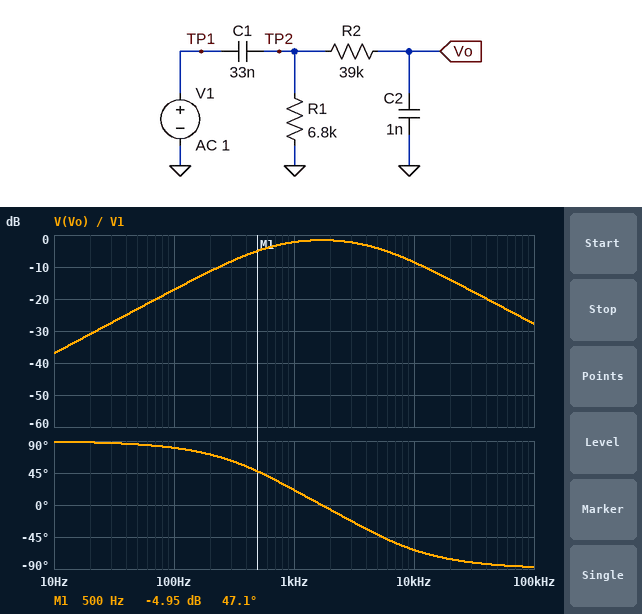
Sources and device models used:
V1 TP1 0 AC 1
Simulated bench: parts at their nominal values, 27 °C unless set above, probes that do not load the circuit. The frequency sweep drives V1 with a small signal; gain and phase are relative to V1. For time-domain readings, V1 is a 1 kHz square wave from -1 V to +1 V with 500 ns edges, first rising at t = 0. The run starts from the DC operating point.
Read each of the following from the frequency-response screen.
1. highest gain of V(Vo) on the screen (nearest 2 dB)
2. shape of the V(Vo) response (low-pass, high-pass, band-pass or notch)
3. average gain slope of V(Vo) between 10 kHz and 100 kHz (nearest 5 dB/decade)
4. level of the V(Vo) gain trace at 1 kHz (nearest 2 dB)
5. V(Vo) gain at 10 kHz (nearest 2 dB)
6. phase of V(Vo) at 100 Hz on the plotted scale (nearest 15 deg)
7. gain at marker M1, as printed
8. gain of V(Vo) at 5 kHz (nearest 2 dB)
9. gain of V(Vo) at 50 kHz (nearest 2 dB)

-2 dB
band-pass
-20 dB/decade
-2 dB
-8 dB
75 deg
-4.95 dB
-4 dB
-22 dB
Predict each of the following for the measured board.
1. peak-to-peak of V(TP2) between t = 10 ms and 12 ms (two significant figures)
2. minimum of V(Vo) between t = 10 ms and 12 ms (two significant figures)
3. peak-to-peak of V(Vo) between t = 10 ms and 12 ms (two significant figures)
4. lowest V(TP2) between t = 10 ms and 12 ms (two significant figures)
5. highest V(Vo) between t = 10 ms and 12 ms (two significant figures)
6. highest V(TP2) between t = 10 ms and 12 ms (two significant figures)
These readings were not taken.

3.6 V
-1.2 V
2.4 V
-1.8 V
1.2 V
1.8 V
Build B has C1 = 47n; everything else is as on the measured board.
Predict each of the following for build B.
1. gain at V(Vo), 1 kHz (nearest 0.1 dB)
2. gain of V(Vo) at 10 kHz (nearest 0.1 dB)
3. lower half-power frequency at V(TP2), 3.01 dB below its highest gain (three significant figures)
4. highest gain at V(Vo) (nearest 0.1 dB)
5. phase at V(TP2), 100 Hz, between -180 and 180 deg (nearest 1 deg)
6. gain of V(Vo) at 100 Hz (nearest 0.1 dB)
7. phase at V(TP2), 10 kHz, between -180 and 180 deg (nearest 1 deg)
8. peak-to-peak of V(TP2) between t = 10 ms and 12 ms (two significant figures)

-1.4 dB
-8.5 dB
510 Hz
-1.2 dB
78 deg
-14.1 dB
3 deg
3.3 V
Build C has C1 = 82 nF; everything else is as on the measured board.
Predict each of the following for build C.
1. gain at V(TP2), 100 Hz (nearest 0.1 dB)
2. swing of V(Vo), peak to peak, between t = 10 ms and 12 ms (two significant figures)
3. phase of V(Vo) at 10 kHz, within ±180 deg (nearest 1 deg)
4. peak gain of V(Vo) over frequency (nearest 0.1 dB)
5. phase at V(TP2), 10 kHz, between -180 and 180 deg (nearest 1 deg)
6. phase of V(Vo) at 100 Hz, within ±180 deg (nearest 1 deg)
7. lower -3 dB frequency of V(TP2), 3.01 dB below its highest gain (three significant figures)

-9.6 dB
2.2 V
-66 deg
-0.7 dB
2 deg
69 deg
289 Hz
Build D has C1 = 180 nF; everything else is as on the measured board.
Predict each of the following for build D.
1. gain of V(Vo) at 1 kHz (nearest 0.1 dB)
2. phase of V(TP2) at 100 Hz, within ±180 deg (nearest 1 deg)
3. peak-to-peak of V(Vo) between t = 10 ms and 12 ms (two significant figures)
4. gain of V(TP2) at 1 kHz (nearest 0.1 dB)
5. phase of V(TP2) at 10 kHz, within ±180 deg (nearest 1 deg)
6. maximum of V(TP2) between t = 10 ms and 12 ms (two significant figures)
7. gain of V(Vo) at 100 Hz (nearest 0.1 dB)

-0.4 dB
52 deg
2.1 V
-0.1 dB
1 deg
1.2 V
-4.3 dB
